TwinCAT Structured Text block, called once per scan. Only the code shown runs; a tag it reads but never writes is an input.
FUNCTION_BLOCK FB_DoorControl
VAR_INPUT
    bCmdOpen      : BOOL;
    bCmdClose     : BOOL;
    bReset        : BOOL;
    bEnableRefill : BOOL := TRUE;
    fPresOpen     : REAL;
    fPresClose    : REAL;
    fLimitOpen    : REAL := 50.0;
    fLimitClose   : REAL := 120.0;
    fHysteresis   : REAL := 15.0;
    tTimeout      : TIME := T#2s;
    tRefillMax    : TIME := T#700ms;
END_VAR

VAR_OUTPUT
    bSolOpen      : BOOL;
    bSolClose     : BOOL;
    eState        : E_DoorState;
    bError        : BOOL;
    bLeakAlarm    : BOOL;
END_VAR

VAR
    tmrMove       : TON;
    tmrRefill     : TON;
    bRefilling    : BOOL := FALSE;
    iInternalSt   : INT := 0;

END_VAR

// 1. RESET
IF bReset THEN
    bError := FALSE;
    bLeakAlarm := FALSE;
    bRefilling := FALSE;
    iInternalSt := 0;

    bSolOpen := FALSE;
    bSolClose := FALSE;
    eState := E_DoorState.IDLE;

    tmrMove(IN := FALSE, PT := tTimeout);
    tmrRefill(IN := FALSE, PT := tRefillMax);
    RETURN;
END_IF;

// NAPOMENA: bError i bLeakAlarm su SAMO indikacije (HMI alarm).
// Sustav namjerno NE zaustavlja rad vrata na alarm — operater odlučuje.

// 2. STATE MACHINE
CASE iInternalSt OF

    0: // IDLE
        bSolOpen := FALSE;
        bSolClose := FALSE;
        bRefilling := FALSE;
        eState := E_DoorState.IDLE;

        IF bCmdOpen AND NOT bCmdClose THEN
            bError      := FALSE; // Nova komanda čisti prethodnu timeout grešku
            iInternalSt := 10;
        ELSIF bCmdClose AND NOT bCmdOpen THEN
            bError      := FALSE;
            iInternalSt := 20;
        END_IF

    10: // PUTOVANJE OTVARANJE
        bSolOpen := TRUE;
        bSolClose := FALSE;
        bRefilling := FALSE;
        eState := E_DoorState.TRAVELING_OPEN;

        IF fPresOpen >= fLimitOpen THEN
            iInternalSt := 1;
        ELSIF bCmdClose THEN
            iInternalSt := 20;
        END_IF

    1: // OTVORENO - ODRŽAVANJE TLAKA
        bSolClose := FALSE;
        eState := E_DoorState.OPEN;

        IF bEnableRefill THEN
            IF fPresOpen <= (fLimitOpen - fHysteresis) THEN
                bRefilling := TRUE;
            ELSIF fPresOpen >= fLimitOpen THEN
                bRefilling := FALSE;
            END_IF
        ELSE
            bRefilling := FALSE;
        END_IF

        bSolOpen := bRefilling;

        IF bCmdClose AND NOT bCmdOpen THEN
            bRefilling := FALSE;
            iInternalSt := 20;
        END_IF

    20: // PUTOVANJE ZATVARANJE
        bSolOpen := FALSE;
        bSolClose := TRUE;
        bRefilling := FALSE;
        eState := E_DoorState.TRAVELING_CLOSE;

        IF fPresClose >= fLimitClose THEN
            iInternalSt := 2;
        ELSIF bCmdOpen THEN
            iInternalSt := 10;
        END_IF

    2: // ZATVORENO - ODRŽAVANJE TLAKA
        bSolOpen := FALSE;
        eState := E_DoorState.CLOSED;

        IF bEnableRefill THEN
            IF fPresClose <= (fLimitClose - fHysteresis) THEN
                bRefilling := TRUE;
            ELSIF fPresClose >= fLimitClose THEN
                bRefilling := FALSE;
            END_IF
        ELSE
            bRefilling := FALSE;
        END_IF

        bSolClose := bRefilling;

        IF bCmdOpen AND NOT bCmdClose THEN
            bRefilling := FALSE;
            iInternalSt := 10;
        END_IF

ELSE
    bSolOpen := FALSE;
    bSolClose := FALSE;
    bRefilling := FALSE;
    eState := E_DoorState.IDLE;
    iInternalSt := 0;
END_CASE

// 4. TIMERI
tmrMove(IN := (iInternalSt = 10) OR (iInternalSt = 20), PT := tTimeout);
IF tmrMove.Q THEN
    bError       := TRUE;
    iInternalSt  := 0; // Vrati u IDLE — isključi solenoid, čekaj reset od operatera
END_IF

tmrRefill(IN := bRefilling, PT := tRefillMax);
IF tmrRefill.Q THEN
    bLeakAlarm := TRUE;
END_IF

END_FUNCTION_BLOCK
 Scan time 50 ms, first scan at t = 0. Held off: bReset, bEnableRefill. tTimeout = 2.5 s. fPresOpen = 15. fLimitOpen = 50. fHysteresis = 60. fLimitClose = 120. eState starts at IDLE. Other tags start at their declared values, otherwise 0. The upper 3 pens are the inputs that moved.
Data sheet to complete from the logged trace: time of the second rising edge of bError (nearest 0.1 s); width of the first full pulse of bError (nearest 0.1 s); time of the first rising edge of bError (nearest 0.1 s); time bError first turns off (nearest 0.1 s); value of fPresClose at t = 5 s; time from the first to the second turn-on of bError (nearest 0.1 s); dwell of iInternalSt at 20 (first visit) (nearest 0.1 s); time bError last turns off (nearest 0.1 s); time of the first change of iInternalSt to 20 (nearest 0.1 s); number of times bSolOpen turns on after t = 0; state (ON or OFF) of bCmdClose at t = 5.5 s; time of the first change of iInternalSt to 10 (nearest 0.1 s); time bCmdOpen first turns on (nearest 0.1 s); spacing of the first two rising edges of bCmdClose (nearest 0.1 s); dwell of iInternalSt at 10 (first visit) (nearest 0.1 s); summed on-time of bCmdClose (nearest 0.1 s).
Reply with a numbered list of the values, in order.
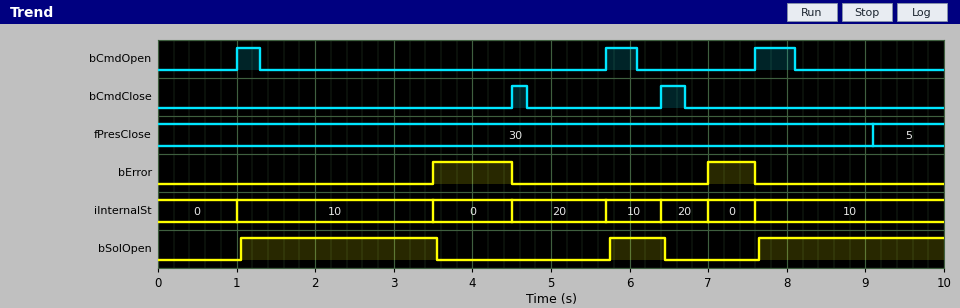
1. 7.0 s
2. 1.0 s
3. 3.5 s
4. 4.5 s
5. 30
6. 3.5 s
7. 1.2 s
8. 7.6 s
9. 4.5 s
10. 3
11. OFF
12. 1.0 s
13. 1.0 s
14. 1.9 s
15. 2.5 s
16. 0.5 s
